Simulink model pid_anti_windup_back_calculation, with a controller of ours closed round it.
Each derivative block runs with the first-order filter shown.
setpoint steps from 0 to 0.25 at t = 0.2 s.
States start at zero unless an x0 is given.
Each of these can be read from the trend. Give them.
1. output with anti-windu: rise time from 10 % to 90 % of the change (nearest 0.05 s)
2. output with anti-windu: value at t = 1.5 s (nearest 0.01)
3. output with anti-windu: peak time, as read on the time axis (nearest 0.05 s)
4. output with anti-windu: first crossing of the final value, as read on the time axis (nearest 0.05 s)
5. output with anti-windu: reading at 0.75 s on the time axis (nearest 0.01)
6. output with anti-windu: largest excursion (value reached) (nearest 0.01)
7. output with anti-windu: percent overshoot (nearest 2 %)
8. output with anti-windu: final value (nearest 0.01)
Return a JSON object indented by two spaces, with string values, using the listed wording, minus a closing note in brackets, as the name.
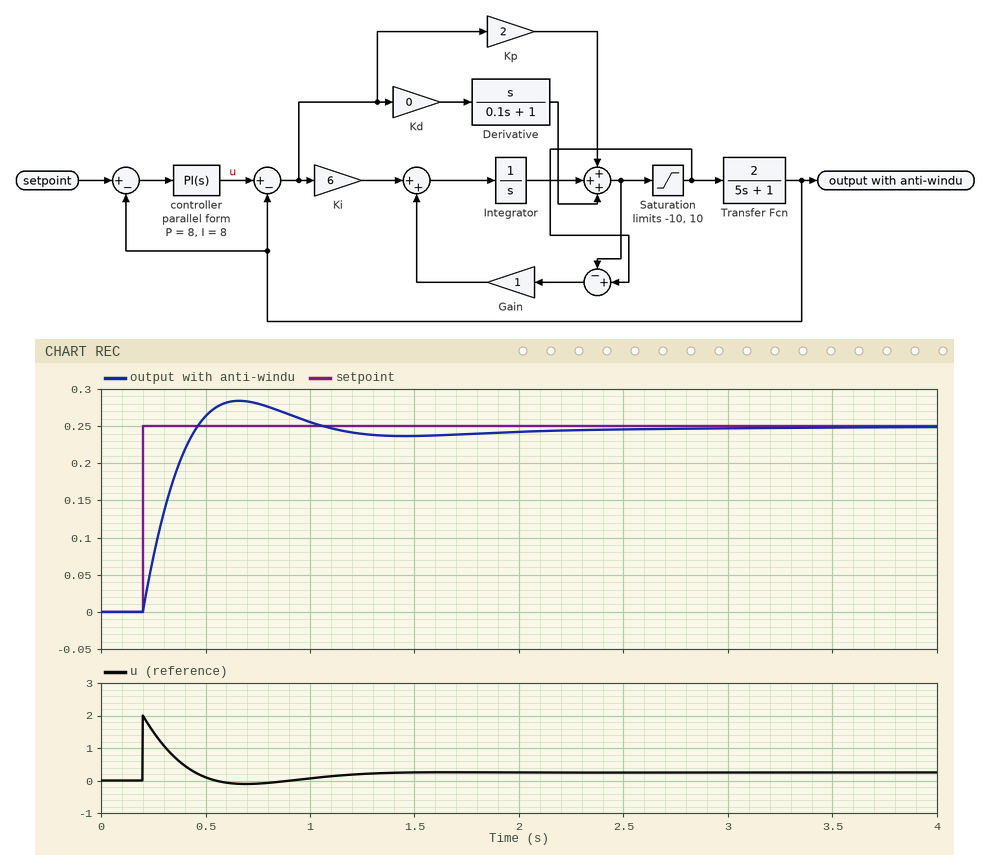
{
  "output with anti-windu: rise time from 10 % to 90 % of the change": "0.20 s",
  "output with anti-windu: value at t = 1.5 s": "0.24",
  "output with anti-windu: peak time, as read on the time axis": "0.65 s",
  "output with anti-windu: first crossing of the final value, as read on the time axis": "0.45 s",
  "output with anti-windu: reading at 0.75 s on the time axis": "0.28",
  "output with anti-windu: largest excursion (value reached)": "0.28",
  "output with anti-windu: percent overshoot": "14 %",
  "output with anti-windu: final value": "0.25"
}
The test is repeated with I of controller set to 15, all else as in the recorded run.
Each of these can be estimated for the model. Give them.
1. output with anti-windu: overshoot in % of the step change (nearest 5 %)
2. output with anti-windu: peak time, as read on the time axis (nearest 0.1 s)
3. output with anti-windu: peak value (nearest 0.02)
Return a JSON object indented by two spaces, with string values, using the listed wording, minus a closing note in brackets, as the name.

{
  "output with anti-windu: overshoot in % of the step change": "20 %",
  "output with anti-windu: peak time, as read on the time axis": "0.6 s",
  "output with anti-windu: peak value": "0.30"
}
